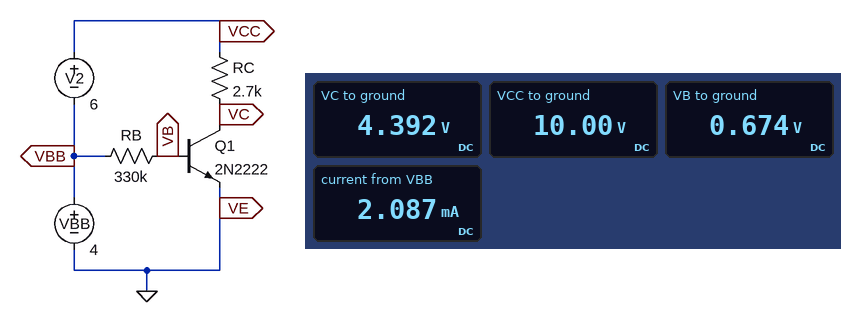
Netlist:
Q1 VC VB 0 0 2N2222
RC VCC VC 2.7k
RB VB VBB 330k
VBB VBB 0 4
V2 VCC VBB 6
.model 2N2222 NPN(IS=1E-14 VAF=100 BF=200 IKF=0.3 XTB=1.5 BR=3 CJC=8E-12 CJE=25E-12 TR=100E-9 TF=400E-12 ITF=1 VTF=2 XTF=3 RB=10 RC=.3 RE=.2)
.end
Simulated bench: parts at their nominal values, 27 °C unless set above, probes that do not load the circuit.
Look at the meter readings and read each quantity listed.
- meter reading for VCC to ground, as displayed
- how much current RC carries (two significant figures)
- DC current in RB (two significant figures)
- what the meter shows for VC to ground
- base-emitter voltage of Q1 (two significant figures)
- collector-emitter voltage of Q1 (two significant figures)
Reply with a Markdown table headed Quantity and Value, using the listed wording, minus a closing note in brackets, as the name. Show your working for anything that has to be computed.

| Quantity | Value |
|---|---|
| meter reading for VCC to ground, as displayed | 10.00 V |
| how much current RC carries | (10 V - 4.392 V) / 2.7 kΩ = 2.1 mA |
| DC current in RB | (4 V - 674 mV) / 330 kΩ = 10 µA |
| what the meter shows for VC to ground | 4.392 V |
| base-emitter voltage of Q1 | 674 mV = 670 mV |
| collector-emitter voltage of Q1 | 4.392 V = 4.4 V |
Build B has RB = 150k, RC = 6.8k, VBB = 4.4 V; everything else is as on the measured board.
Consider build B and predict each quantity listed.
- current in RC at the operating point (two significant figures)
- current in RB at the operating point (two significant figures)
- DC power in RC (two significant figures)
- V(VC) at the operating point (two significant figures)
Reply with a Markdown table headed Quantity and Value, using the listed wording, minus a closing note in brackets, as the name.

| Quantity | Value |
|---|---|
| current in RC at the operating point | 1.5 mA |
| current in RB at the operating point | 25 µA |
| DC power in RC | 16 mW |
| V(VC) at the operating point | 90 mV |
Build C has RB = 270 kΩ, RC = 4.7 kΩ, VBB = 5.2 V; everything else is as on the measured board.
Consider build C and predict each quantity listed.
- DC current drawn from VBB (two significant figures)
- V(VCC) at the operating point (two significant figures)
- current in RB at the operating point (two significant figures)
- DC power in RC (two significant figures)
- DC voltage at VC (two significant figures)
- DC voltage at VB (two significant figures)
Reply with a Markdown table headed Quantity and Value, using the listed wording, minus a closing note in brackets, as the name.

| Quantity | Value |
|---|---|
| DC current drawn from VBB | 2.4 mA |
| V(VCC) at the operating point | 11 V |
| current in RB at the operating point | 17 µA |
| DC power in RC | 26 mW |
| DC voltage at VC | 130 mV |
| DC voltage at VB | 680 mV |
